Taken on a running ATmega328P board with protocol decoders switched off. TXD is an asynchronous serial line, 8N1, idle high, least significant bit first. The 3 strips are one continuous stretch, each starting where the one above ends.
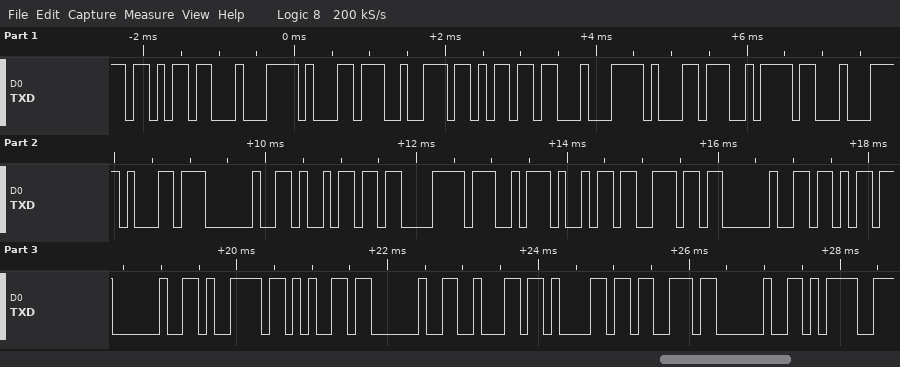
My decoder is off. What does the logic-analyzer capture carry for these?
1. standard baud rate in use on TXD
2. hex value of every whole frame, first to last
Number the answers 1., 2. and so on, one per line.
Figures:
1. 9600 baud
2. 0x6B 0xC4 0xB1 0x72 0x6D 0xC4 0xB1 0x7A 0xC4 0xB1 0x20 0x69 0xC3 0xA7 0x69 0x6E 0x20 0x6B 0x20 0x79 0x65 0x20 0x62 0x61 0x73 0x20 0x3D
